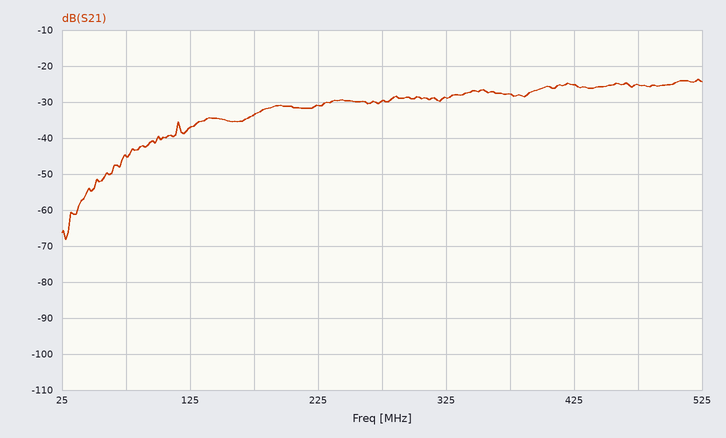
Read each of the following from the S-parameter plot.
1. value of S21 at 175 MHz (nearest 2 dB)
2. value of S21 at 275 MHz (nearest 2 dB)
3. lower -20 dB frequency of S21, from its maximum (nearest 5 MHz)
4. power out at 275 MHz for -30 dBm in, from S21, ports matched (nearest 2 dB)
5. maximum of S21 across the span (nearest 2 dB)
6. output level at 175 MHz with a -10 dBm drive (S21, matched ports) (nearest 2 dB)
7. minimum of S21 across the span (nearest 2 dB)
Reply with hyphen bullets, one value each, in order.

- -34 dB
- -30 dB
- 80 MHz
- -60 dBm
- -24 dB
- -44 dBm
- -68 dB
